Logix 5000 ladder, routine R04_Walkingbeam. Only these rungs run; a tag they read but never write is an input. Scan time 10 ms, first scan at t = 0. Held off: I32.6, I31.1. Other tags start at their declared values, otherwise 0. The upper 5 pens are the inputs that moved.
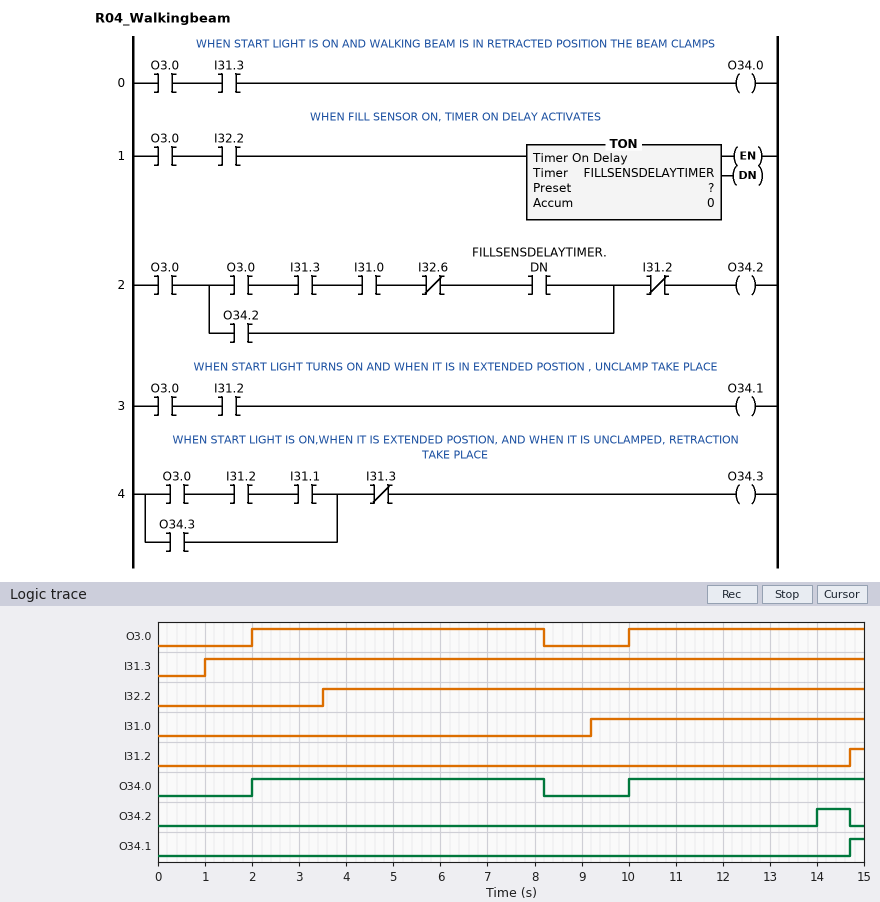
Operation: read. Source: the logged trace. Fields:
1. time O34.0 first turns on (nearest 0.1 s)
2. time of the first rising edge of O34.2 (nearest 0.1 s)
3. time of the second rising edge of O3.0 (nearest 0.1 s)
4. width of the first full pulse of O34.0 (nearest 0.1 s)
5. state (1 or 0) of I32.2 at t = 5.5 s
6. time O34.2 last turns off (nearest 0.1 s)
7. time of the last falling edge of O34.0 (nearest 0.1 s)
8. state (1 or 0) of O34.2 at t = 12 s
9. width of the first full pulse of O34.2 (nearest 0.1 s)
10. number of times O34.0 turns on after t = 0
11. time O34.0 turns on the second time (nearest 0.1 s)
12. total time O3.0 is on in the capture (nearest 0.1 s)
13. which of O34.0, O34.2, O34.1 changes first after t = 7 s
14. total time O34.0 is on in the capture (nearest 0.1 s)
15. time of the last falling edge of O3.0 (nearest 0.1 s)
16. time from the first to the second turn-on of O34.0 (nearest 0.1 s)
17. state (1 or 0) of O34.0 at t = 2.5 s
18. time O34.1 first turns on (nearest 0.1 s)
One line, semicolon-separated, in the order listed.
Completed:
2.0 s; 14.0 s; 10.0 s; 6.2 s; 1; 14.7 s; 8.2 s; 0; 0.7 s; 2; 10.0 s; 11.2 s; O34.0; 11.2 s; 8.2 s; 8.0 s; 1; 14.7 s
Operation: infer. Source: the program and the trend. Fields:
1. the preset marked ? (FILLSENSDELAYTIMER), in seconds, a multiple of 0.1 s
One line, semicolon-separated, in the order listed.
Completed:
4.0 s
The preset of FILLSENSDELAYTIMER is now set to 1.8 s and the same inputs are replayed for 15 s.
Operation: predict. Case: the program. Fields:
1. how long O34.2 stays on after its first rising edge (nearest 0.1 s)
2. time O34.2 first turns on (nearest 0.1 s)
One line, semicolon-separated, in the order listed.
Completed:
2.9 s; 11.8 s
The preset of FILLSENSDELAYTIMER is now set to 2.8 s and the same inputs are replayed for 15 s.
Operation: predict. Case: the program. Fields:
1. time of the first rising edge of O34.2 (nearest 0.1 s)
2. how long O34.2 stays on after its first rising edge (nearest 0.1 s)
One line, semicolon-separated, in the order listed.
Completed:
12.8 s; 1.9 s
